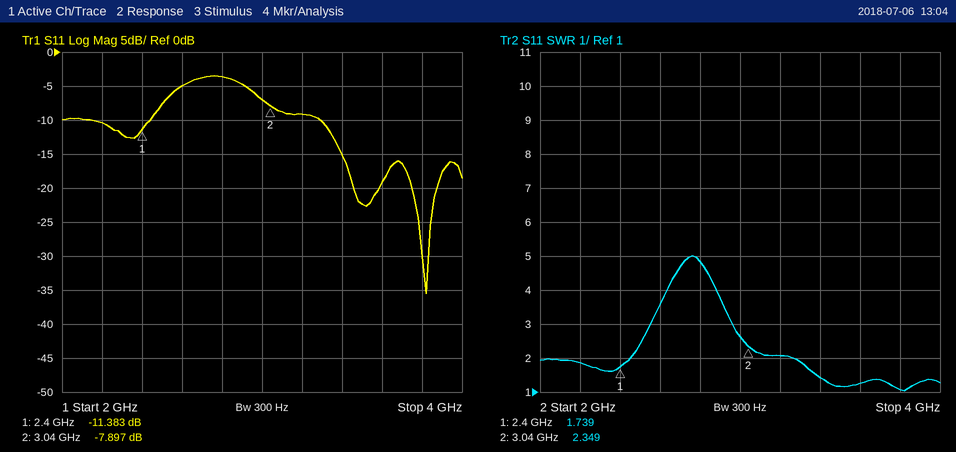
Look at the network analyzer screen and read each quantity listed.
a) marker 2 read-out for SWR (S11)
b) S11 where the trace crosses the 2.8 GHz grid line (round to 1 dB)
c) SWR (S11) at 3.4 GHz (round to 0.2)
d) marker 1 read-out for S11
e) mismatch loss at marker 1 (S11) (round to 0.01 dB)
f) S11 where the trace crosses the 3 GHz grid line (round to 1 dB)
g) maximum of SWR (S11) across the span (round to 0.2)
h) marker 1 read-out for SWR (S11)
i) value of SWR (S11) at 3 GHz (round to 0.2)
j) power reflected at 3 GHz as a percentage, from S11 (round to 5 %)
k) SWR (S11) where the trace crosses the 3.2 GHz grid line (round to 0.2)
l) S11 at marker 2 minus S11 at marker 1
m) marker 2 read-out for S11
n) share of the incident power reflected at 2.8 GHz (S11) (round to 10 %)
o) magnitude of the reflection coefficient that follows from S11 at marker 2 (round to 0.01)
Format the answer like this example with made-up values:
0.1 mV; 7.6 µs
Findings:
2.349; -4 dB; 1.4; -11.383 dB; 0.33 dB; -7 dB; 5.0; 1.739; 2.6; 20 %; 2.0; 3.486 dB; -7.897 dB; 40 %; 0.40
